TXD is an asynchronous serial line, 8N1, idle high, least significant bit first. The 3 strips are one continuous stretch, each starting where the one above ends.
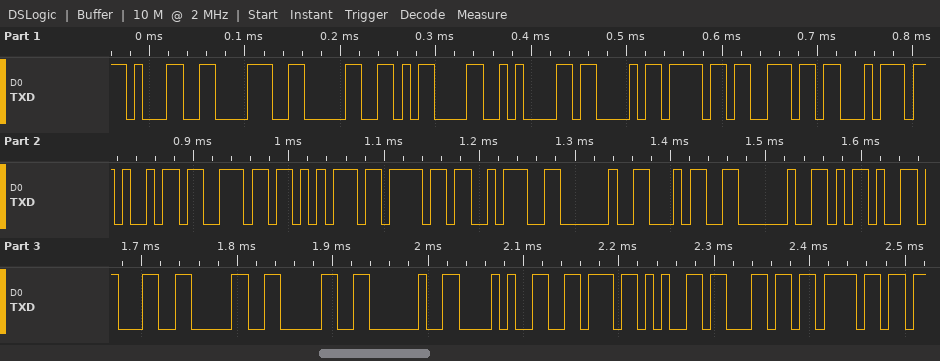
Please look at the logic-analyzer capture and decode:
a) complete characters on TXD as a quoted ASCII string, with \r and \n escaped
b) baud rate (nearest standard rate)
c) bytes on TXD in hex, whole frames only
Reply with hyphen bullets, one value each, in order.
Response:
- "180\r\nContinuo: 4 -100 (velo"
- 115200 baud
- 31 38 30 0D 0A 43 6F 6E 74 69 6E 75 6F 3A 20 34 20 2D 31 30 30 20 28 76 65 6C 6F
